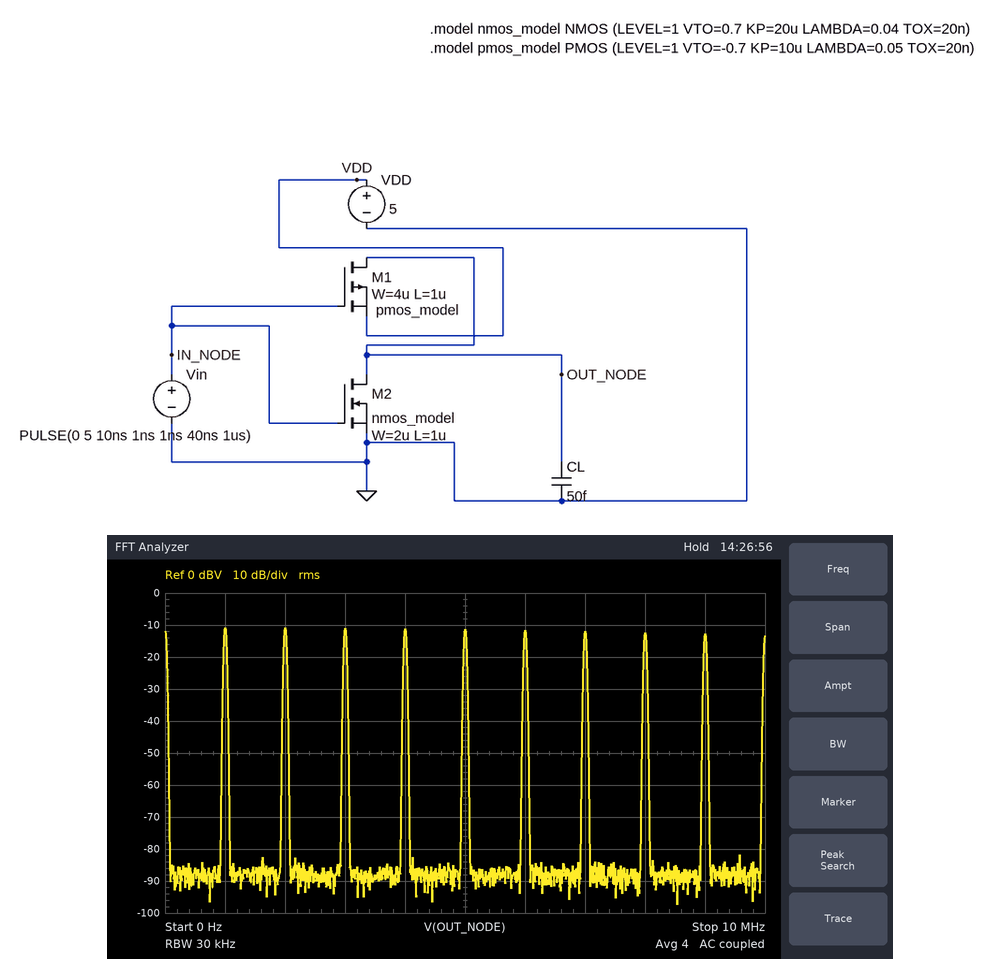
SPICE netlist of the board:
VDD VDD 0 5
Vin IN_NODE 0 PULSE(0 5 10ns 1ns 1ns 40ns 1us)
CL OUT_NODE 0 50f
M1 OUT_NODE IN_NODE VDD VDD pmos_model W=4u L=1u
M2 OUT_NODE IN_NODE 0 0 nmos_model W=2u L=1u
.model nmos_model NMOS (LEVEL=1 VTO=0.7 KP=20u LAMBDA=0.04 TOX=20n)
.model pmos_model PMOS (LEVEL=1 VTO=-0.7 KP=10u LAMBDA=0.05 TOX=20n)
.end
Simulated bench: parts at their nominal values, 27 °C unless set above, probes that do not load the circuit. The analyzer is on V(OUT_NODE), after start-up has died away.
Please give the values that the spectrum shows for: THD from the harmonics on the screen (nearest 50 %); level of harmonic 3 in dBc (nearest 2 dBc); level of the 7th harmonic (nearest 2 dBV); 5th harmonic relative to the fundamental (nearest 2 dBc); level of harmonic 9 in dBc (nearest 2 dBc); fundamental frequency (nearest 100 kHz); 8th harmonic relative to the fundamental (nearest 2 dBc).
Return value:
250 %
0 dBc
-12 dBV
0 dBc
-2 dBc
1.0 MHz
-2 dBc
